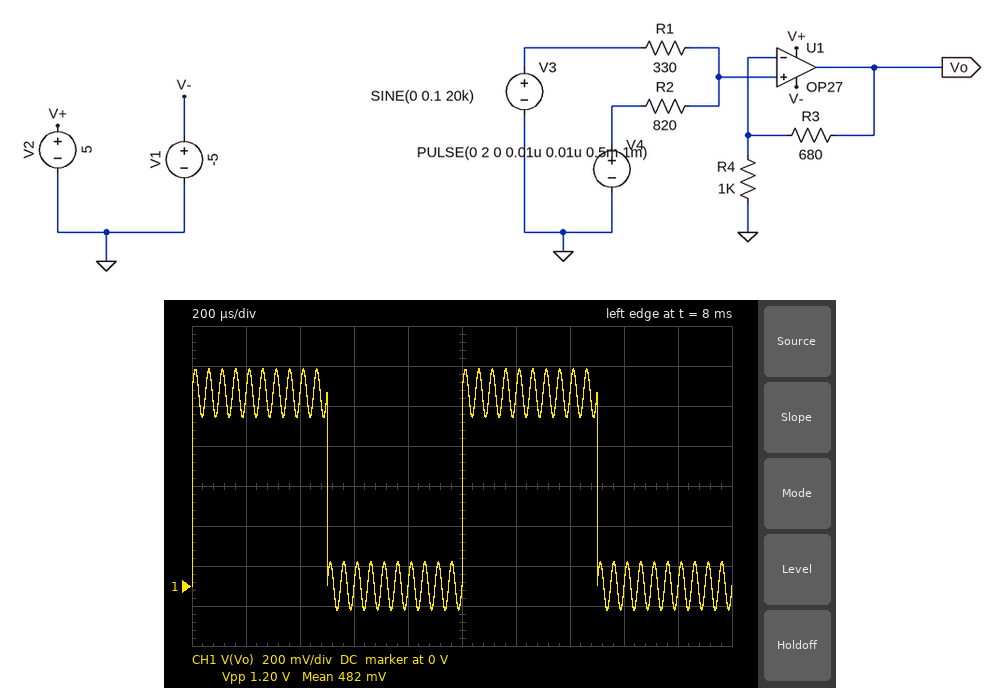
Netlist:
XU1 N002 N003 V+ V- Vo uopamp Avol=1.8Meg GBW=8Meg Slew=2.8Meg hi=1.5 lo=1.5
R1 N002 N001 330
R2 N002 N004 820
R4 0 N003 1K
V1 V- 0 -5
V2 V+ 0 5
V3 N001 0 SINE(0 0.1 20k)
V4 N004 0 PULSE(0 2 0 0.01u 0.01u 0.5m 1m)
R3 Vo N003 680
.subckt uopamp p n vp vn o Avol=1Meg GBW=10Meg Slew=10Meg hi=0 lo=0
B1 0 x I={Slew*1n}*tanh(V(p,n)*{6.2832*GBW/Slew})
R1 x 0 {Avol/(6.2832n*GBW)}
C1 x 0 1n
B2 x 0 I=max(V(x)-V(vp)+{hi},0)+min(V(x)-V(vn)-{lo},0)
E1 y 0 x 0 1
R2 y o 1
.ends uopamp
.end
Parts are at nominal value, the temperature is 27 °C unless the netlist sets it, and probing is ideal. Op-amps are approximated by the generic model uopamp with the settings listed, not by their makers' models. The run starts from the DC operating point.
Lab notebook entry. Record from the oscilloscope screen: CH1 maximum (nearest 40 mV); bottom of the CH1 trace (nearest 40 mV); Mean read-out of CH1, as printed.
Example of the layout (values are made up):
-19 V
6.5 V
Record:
1.08 V
-120 mV
482 mV
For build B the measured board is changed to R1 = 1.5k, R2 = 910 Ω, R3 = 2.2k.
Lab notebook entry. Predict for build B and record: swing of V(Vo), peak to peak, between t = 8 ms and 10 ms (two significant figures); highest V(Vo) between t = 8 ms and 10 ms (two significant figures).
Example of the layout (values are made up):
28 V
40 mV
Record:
3.6 V
3.5 V
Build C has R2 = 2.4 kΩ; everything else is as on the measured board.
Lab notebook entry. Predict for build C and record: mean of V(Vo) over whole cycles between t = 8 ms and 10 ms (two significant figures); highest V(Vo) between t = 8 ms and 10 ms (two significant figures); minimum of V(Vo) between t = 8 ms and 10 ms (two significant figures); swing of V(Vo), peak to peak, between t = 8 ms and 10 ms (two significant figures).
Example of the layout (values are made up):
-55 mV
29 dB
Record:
200 mV
550 mV
-150 mV
700 mV
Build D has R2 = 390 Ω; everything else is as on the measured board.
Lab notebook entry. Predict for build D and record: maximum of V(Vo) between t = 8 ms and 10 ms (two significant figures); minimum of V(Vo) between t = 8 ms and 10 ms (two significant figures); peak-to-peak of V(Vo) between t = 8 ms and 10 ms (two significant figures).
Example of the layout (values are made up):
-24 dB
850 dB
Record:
1.6 V
-91 mV
1.7 V
